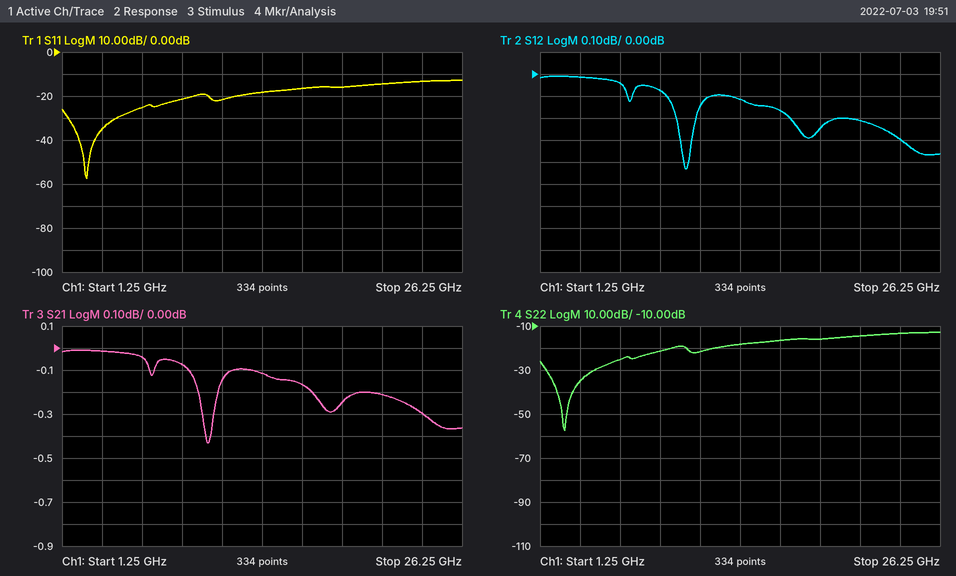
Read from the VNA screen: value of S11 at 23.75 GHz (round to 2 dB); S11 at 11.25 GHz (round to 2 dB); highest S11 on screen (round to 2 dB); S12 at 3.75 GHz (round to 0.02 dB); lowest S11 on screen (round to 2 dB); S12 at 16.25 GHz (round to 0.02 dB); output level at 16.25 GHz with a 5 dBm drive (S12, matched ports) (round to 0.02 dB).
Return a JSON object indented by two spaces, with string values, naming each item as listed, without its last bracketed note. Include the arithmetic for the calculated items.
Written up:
{
  "value of S11 at 23.75 GHz": "-14 dB",
  "S11 at 11.25 GHz": "-22 dB",
  "highest S11 on screen": "-12 dB",
  "S12 at 3.75 GHz": "-0.02 dB",
  "lowest S11 on screen": "-58 dB",
  "S12 at 16.25 GHz": "-0.16 dB",
  "output level at 16.25 GHz with a 5 dBm drive (S12, matched ports)": "5 dBm + (-0.16 dB) = 4.84 dBm"
}
